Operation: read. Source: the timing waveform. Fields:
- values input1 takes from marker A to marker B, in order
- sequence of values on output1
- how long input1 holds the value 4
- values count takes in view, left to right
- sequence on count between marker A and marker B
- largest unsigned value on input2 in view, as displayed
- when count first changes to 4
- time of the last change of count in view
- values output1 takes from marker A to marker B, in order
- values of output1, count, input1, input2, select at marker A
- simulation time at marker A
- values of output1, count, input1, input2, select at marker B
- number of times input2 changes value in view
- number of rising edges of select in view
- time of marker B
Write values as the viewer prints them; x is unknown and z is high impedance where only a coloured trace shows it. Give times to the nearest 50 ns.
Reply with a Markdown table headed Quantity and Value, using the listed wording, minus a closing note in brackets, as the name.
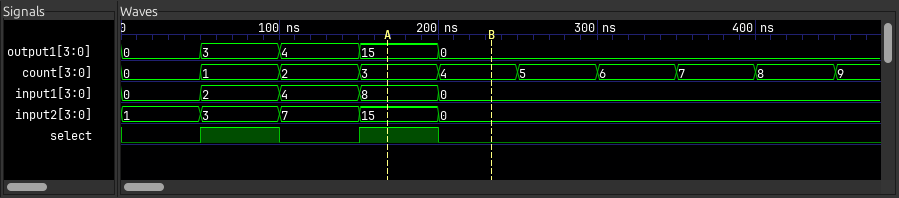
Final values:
| Quantity | Value |
|---|---|
| values input1 takes from marker A to marker B, in order | 8, 0 |
| sequence of values on output1 | 0, 3, 4, 15, 0 |
| how long input1 holds the value 4 | 50 ns |
| values count takes in view, left to right | 0, 1, 2, 3, 4, 5, 6, 7, 8, 9 |
| sequence on count between marker A and marker B | 3, 4 |
| largest unsigned value on input2 in view, as displayed | 15 |
| when count first changes to 4 | 200 ns |
| time of the last change of count in view | 450 ns |
| values output1 takes from marker A to marker B, in order | 15, 0 |
| values of output1, count, input1, input2, select at marker A | output1=15, count=3, input1=8, input2=15, select=1 |
| simulation time at marker A | 150 ns |
| values of output1, count, input1, input2, select at marker B | output1=0, count=4, input1=0, input2=0, select=0 |
| number of times input2 changes value in view | 4 |
| number of rising edges of select in view | 2 |
| time of marker B | 250 ns |
